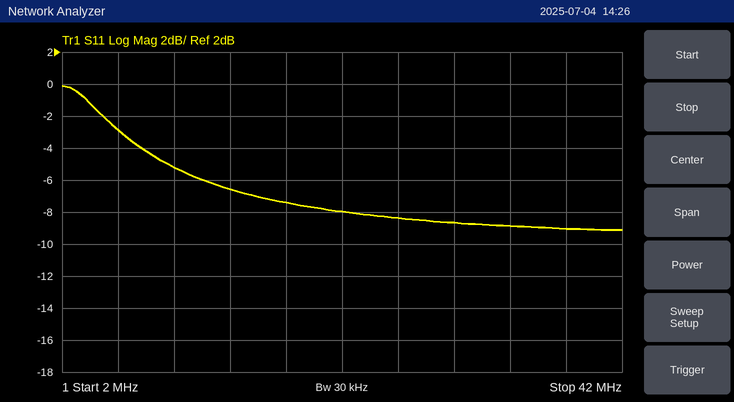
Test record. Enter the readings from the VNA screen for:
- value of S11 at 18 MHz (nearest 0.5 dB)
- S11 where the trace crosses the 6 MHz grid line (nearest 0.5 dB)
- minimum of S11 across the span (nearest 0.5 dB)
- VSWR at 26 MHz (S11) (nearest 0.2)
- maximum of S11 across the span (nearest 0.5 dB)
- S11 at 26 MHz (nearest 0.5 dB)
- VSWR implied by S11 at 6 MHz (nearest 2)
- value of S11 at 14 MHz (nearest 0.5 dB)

-7.5 dB
-3.0 dB
-9.0 dB
2.2
0.0 dB
-8.5 dB
6
-6.5 dB
